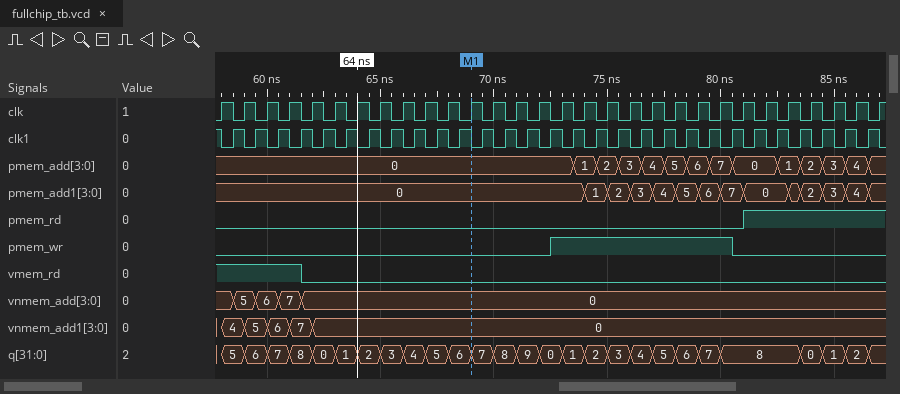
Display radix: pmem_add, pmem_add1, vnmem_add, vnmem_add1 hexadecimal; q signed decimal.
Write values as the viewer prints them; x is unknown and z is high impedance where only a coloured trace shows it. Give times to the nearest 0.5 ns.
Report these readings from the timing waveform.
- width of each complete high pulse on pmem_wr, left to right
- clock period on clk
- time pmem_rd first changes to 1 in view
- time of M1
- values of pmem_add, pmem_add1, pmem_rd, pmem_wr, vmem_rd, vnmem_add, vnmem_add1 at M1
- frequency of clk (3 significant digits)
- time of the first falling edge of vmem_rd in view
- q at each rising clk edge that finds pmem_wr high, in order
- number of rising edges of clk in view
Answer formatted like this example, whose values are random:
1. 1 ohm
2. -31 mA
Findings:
1. 8 ns
2. 1 ns
3. 81 ns
4. 69 ns
5. pmem_add=0, pmem_add1=0, pmem_rd=0, pmem_wr=0, vmem_rd=0, vnmem_add=0, vnmem_add1=0
6. 1.00 GHz
7. 61.5 ns
8. 0, 1, 2, 3, 4, 5, 6, 7
9. 30
